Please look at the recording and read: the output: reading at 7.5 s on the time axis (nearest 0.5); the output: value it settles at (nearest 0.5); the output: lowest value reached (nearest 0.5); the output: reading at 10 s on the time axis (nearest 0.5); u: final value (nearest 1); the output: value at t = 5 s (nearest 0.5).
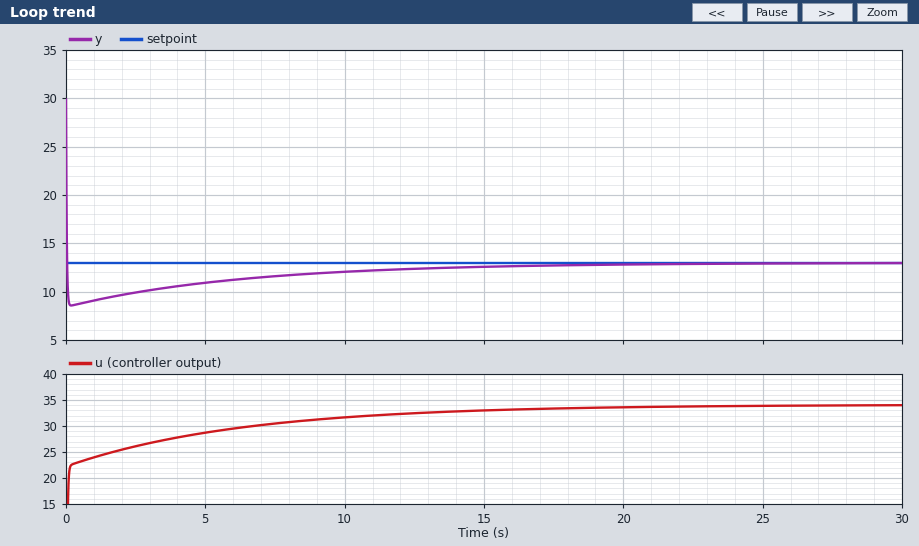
11.5
13.0
8.5
12.0
34
11.0
